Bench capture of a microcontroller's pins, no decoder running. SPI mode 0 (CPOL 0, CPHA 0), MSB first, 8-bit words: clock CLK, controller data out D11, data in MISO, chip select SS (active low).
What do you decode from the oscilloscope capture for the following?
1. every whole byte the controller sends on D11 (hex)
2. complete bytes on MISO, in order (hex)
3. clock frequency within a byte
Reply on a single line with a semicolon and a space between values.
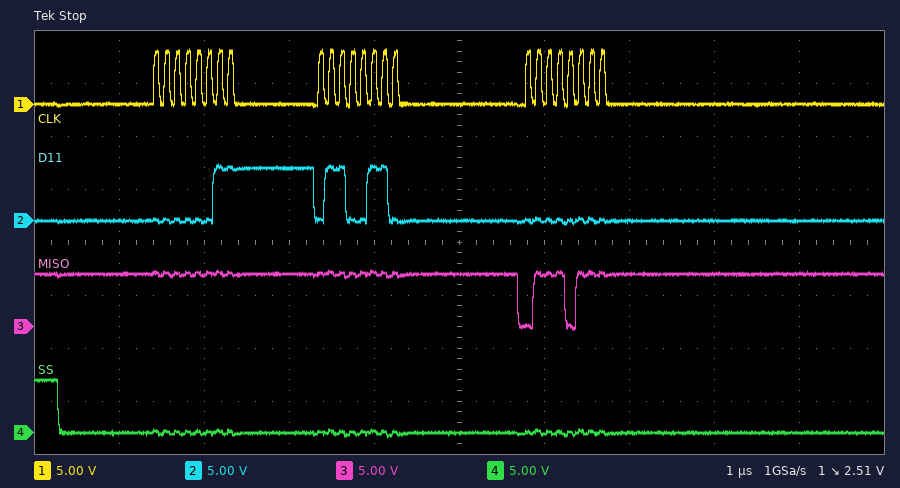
03 66 00; FF FF 77; 8 MHz
